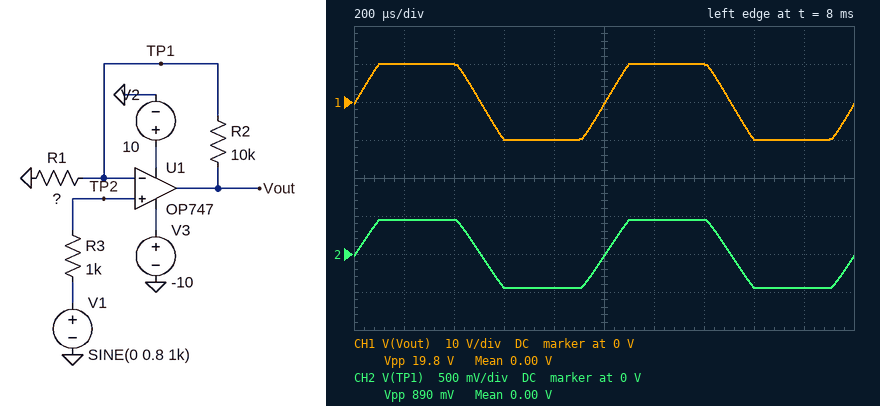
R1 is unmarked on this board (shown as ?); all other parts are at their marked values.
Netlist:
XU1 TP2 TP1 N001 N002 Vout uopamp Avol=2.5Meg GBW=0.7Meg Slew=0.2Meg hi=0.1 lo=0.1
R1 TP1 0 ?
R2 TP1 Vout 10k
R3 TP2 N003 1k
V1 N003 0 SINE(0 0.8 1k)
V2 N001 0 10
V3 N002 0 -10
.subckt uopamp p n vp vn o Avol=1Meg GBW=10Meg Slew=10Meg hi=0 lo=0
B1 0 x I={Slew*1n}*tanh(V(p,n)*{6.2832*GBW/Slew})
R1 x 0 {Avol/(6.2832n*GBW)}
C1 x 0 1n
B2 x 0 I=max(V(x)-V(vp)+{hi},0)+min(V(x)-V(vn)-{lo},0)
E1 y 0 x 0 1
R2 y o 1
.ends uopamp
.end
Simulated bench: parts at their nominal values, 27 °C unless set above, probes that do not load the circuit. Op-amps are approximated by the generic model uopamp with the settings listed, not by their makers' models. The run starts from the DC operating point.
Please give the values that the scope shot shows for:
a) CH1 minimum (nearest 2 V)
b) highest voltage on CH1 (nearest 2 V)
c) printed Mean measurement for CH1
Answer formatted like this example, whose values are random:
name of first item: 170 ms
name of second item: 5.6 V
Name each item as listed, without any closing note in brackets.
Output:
CH1 minimum: -10 V
highest voltage on CH1: 10 V
printed Mean measurement for CH1: 0.00 V
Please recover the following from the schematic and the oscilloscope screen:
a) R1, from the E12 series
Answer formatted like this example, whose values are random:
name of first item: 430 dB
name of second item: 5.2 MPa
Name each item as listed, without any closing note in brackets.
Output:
R1, from the E12 series: 470 Ω
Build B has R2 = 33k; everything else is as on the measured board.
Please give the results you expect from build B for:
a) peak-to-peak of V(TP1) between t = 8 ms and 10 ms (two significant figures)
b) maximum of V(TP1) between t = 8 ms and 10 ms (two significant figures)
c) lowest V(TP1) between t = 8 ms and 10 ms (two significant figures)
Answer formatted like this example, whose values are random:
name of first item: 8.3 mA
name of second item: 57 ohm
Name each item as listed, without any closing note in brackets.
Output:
peak-to-peak of V(TP1) between t = 8 ms and 10 ms: 280 mV
maximum of V(TP1) between t = 8 ms and 10 ms: 140 mV
lowest V(TP1) between t = 8 ms and 10 ms: -140 mV
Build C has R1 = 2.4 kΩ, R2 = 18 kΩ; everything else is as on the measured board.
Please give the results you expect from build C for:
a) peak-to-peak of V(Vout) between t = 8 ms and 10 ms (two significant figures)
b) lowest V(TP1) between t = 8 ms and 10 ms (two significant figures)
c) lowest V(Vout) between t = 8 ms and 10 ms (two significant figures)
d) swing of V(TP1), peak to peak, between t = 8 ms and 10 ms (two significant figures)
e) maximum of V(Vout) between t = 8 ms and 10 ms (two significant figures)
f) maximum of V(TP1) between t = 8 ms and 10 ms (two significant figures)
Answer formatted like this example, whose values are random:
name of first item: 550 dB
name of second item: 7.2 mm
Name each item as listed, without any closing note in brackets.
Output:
peak-to-peak of V(Vout) between t = 8 ms and 10 ms: 14 V
lowest V(TP1) between t = 8 ms and 10 ms: -800 mV
lowest V(Vout) between t = 8 ms and 10 ms: -6.8 V
swing of V(TP1), peak to peak, between t = 8 ms and 10 ms: 1.6 V
maximum of V(Vout) between t = 8 ms and 10 ms: 6.8 V
maximum of V(TP1) between t = 8 ms and 10 ms: 800 mV
